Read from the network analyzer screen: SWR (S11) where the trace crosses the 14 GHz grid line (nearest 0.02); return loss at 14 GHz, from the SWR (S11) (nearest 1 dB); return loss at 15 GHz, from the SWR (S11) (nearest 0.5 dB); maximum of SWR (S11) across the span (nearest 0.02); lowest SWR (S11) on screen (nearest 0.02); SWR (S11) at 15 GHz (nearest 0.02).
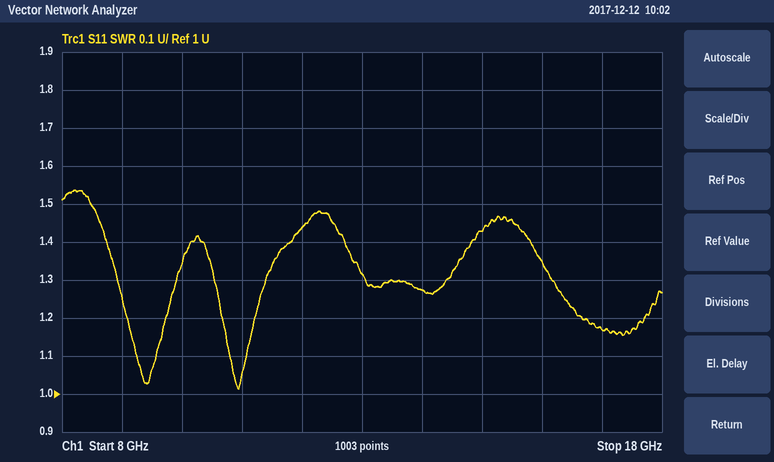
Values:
1.28
18 dB
15.0 dB
1.54
1.02
1.42
